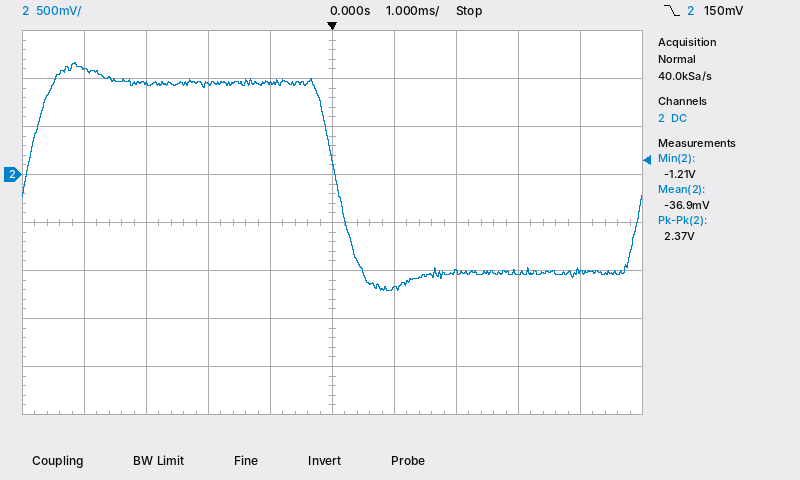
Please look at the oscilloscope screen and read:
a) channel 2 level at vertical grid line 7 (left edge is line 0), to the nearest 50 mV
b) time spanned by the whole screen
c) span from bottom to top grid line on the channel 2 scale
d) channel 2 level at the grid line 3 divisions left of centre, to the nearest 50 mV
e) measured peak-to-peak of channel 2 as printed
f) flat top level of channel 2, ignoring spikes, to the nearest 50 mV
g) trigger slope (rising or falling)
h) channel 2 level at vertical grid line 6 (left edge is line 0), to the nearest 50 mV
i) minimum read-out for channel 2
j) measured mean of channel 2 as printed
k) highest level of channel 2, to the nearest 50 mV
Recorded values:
-1.00 V
10 ms
4 V
950 mV
2.37 V
950 mV
falling
-1.20 V
-1.21 V
-36.9 mV
1.15 V
